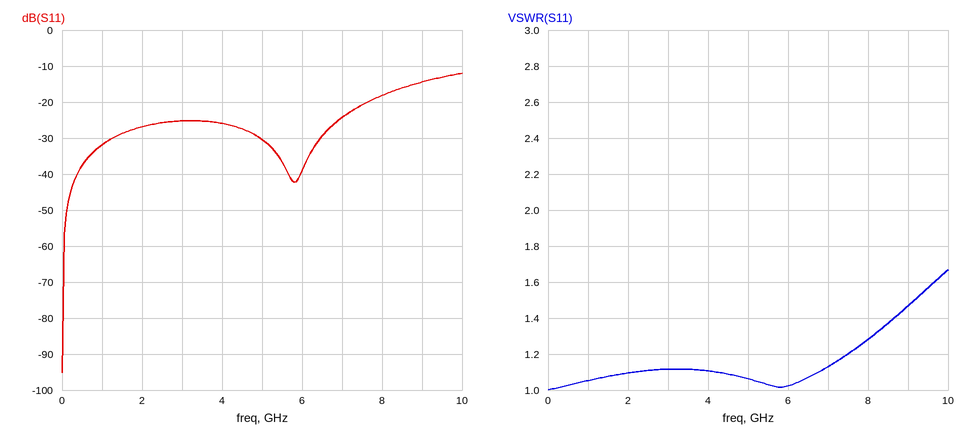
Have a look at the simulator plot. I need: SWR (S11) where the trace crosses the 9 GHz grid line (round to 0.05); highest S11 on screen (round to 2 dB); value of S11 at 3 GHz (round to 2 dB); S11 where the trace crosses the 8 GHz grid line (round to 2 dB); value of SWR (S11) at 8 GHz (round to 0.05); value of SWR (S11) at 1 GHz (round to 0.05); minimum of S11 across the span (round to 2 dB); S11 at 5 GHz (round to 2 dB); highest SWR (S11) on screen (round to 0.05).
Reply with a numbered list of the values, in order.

1. 1.45
2. -12 dB
3. -26 dB
4. -18 dB
5. 1.30
6. 1.05
7. -96 dB
8. -30 dB
9. 1.65
